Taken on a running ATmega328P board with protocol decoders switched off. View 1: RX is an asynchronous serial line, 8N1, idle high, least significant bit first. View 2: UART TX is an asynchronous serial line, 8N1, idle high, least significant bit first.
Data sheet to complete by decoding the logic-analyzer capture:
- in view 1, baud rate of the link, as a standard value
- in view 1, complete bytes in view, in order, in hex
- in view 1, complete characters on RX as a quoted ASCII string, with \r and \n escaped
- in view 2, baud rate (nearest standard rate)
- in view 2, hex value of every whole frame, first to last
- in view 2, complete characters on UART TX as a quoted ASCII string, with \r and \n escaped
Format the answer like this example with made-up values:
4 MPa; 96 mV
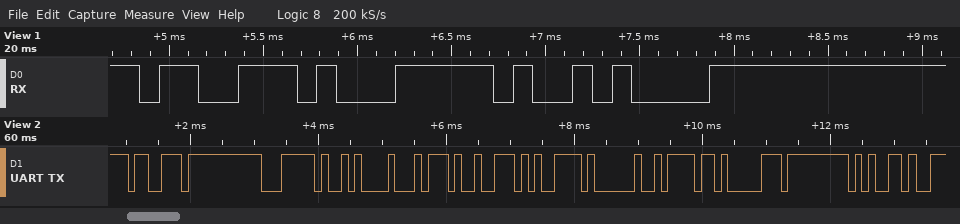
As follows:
9600 baud; 73 7C 0A; "s|\n"; 9600 baud; 0x73 0x7C 0x0A 0x74 0x72 0x79 0x20 0x6F 0x70 0x65; "s|\ntry ope"
